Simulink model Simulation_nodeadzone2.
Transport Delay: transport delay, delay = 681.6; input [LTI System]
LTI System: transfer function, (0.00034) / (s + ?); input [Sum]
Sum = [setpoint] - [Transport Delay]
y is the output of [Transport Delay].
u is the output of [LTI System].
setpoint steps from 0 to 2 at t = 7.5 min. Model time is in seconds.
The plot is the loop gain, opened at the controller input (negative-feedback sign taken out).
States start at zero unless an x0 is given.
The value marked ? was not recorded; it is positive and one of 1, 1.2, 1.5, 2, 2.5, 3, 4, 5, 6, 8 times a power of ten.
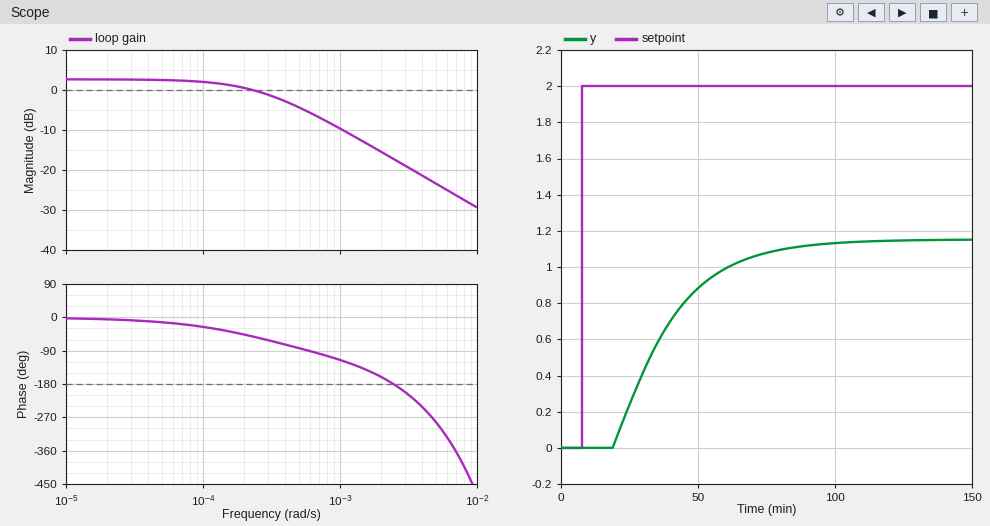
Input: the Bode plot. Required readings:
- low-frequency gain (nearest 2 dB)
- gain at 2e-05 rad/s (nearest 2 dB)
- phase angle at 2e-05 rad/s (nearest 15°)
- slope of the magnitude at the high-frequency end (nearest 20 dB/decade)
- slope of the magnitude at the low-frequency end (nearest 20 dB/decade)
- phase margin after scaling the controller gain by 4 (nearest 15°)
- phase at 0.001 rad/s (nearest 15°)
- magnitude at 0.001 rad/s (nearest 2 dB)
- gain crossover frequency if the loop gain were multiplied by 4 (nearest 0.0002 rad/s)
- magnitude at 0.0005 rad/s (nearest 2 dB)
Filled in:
2 dB
2 dB
0°
-20 dB/decade
0 dB/decade
45°
-120°
-10 dB
0.0014 rad/s
-4 dB
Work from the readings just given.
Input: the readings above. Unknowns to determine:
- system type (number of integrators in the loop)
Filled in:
0
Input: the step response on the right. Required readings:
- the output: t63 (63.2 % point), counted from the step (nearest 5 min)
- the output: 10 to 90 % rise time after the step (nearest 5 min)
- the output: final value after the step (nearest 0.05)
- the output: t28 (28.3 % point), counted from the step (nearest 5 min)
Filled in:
35 min
45 min
1.15
20 min
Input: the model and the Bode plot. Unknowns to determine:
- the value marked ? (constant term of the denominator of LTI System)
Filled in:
0.00025
